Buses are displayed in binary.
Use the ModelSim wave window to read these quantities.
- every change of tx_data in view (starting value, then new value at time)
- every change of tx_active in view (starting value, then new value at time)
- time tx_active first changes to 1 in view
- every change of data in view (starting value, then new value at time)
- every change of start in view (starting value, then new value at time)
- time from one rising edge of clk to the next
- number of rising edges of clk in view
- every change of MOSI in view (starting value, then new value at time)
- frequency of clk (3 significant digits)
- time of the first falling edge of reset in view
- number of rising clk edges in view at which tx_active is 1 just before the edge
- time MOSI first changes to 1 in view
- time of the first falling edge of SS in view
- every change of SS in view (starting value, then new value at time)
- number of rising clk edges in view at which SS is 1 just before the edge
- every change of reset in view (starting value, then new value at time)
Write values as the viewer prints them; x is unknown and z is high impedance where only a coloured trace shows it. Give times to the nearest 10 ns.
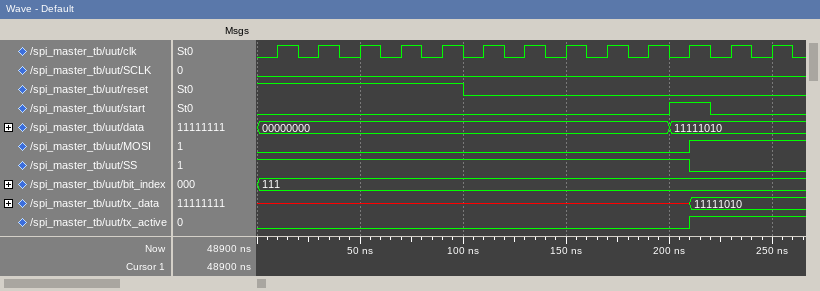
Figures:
x, 11111010 at 210 ns
0, 1 at 210 ns
210 ns
00000000, 11111010 at 200 ns
0, 1 at 200 ns, 0 at 220 ns
20 ns
13
0, 1 at 210 ns
50.0 MHz
100 ns
2
210 ns
210 ns
1, 0 at 210 ns
11
1, 0 at 100 ns
